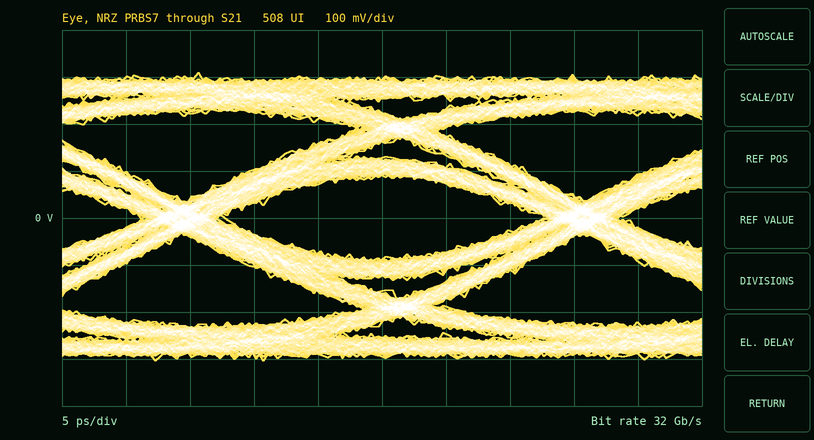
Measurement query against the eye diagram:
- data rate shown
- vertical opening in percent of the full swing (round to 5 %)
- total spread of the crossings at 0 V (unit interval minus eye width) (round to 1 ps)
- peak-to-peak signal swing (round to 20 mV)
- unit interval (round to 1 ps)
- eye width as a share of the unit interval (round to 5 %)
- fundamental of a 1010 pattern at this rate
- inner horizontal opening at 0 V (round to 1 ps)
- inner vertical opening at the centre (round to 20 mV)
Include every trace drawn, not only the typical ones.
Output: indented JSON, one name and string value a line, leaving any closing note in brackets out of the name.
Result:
{
  "data rate shown": "32 Gb/s",
  "vertical opening in percent of the full swing": "30 %",
  "total spread of the crossings at 0 V (unit interval minus eye width)": "6 ps",
  "peak-to-peak signal swing": "620 mV",
  "unit interval": "31 ps",
  "eye width as a share of the unit interval": "80 %",
  "fundamental of a 1010 pattern at this rate": "16 GHz",
  "inner horizontal opening at 0 V": "25 ps",
  "inner vertical opening at the centre": "180 mV"
}
